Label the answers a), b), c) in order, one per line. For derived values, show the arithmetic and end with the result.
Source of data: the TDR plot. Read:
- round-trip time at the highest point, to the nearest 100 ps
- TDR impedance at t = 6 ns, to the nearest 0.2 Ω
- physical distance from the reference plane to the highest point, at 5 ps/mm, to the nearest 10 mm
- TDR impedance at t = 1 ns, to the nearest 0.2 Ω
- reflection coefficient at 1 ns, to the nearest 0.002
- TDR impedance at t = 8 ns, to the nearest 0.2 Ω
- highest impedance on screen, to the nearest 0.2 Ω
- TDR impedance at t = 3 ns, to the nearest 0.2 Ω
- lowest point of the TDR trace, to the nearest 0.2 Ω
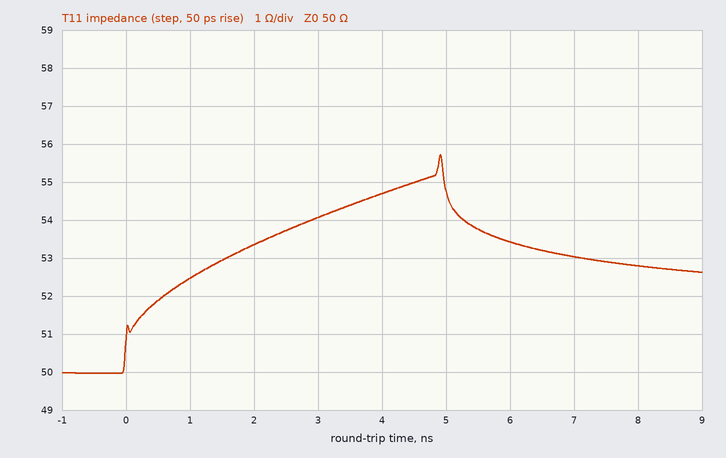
a) 4.9 ns
b) 53.4 Ω
c) 4.9 ns / 2 / 5 ps/mm ≈ 490 mm
d) 52.4 Ω
e) (52.4 − 50)/(52.4 + 50) ≈ +0.0234, so +0.024 to the nearest 0.002
f) 52.8 Ω
g) 55.8 Ω
h) 54.0 Ω
i) 50.0 Ω
